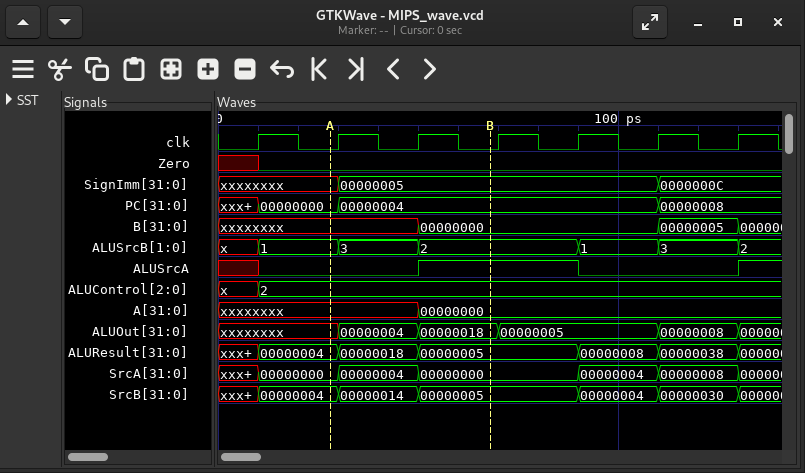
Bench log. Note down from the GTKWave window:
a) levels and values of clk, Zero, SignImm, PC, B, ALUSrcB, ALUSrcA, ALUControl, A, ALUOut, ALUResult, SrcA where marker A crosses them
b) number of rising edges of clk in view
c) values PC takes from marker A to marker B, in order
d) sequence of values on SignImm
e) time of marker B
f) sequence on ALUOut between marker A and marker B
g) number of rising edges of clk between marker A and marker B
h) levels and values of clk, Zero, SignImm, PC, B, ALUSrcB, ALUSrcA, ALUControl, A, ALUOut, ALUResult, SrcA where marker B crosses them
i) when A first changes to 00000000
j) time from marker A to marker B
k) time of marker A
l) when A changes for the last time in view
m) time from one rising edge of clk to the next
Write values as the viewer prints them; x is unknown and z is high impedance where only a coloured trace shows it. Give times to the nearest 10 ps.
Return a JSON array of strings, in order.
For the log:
["clk=0, Zero=0, SignImm=xxxxxxxx, PC=00000000, B=xxxxxxxx, ALUSrcB=1, ALUSrcA=0, ALUControl=2, A=xxxxxxxx, ALUOut=xxxxxxxx, ALUResult=00000004, SrcA=00000000", "7", "00000000, 00000004", "xxxxxxxx, 00000005, 0000000C", "70 ps", "xxxxxxxx, 00000004, 00000018", "2", "clk=0, Zero=0, SignImm=00000005, PC=00000004, B=00000000, ALUSrcB=2, ALUSrcA=1, ALUControl=2, A=00000000, ALUOut=00000018, ALUResult=00000005, SrcA=00000000", "50 ps", "40 ps", "30 ps", "50 ps", "20 ps"]
